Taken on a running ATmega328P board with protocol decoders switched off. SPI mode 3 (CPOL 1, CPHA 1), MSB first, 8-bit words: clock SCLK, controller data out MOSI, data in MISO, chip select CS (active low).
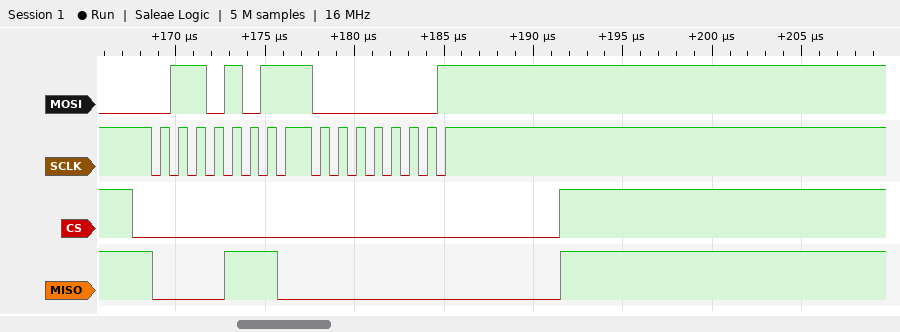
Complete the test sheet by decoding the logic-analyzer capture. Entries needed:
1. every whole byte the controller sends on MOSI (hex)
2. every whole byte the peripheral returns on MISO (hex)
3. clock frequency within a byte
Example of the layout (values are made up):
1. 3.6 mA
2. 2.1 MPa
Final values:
1. 6B 01
2. 0E 00
3. 1 MHz
